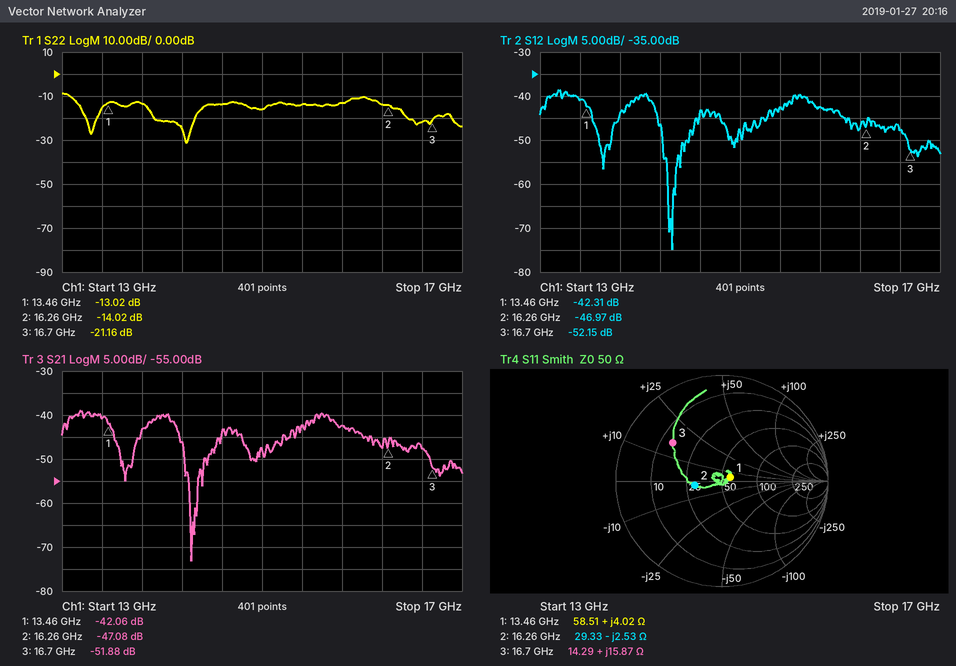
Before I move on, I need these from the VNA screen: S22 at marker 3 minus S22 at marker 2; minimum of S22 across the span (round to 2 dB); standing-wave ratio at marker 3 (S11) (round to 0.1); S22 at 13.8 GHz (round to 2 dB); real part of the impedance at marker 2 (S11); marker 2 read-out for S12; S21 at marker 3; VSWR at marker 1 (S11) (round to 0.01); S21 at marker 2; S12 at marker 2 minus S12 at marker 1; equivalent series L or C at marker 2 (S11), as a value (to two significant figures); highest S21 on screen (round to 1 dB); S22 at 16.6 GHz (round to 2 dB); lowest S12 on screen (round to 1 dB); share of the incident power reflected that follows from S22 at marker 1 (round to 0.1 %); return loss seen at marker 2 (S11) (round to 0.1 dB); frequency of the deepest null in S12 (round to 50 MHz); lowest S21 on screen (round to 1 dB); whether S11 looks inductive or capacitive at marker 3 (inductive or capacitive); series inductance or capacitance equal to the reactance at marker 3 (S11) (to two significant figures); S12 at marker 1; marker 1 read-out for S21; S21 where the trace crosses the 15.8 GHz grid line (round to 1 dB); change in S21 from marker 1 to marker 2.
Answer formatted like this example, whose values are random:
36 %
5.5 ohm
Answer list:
-7.14 dB
-32 dB
3.9
-14 dB
29.33 Ω
-46.97 dB
-51.88 dB
1.19
-47.08 dB
-4.66 dB
3.9 pF
-39 dB
-22 dB
-75 dB
5.0 %
11.6 dB
14.30 GHz
-73 dB
inductive
150 pH
-42.31 dB
-42.06 dB
-42 dB
-5.02 dB
